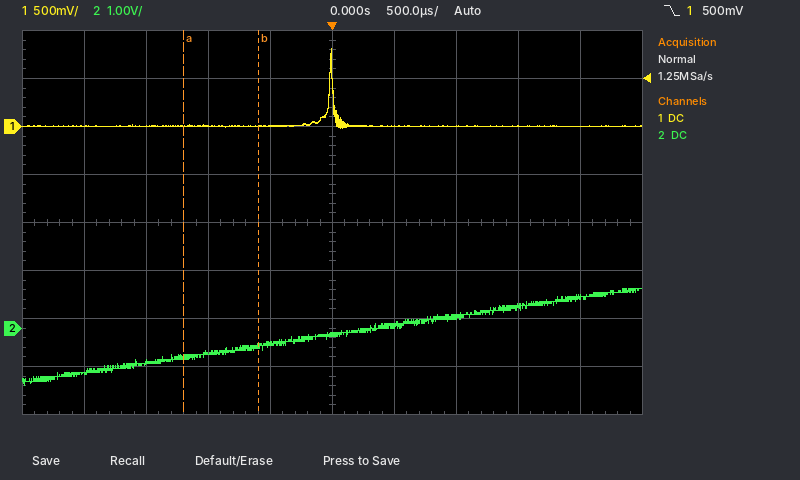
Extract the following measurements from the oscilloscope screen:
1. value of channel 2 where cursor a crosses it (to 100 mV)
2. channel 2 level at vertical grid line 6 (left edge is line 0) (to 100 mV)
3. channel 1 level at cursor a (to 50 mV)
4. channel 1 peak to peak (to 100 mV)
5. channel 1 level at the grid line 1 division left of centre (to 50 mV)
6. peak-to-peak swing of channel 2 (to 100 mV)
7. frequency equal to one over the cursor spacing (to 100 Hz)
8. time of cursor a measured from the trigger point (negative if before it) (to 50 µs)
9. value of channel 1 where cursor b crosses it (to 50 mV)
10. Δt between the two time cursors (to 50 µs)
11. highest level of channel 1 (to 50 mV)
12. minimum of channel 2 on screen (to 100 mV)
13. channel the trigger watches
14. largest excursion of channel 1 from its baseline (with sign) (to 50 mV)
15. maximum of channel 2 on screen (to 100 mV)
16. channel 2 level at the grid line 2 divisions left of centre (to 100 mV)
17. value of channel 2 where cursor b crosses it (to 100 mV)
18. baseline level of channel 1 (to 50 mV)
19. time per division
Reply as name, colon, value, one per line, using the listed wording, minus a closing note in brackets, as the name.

value of channel 2 where cursor a crosses it: -600 mV
channel 2 level at vertical grid line 6 (left edge is line 0): 100 mV
channel 1 level at cursor a: 0 mV
channel 1 peak to peak: 800 mV
channel 1 level at the grid line 1 division left of centre: 0 mV
peak-to-peak swing of channel 2: 2.0 V
frequency equal to one over the cursor spacing: 1.7 kHz
time of cursor a measured from the trigger point (negative if before it): -1.20 ms
value of channel 1 where cursor b crosses it: 0 mV
Δt between the two time cursors: 600 µs
highest level of channel 1: 800 mV
minimum of channel 2 on screen: -1.2 V
channel the trigger watches: channel 1
largest excursion of channel 1 from its baseline (with sign): +800 mV
maximum of channel 2 on screen: 800 mV
channel 2 level at the grid line 2 divisions left of centre: -500 mV
value of channel 2 where cursor b crosses it: -400 mV
baseline level of channel 1: 0 mV
time per division: 500 µs
